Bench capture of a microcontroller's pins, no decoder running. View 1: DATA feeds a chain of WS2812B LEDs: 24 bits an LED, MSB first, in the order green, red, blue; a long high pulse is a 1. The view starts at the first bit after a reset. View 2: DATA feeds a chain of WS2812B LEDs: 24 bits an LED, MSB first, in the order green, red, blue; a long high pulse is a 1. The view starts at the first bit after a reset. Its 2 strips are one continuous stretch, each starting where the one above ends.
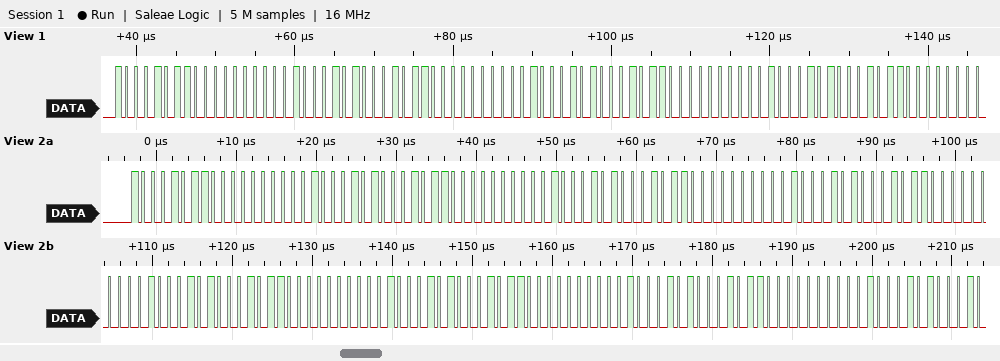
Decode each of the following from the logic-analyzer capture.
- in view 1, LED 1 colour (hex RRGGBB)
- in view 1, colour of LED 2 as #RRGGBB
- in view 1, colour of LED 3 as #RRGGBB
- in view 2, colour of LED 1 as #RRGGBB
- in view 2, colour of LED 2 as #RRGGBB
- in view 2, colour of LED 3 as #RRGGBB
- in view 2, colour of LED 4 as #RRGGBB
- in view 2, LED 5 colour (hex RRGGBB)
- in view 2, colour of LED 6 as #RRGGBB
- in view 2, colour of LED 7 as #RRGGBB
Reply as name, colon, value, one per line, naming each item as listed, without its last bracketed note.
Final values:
in view 1, LED 1 colour: #008B22
in view 1, colour of LED 2 as #RRGGBB: #008B22
in view 1, colour of LED 3 as #RRGGBB: #008B22
in view 2, colour of LED 1 as #RRGGBB: #008B22
in view 2, colour of LED 2 as #RRGGBB: #008B22
in view 2, colour of LED 3 as #RRGGBB: #008B22
in view 2, colour of LED 4 as #RRGGBB: #008B22
in view 2, LED 5 colour: #008B22
in view 2, colour of LED 6 as #RRGGBB: #008B22
in view 2, colour of LED 7 as #RRGGBB: #008B22
